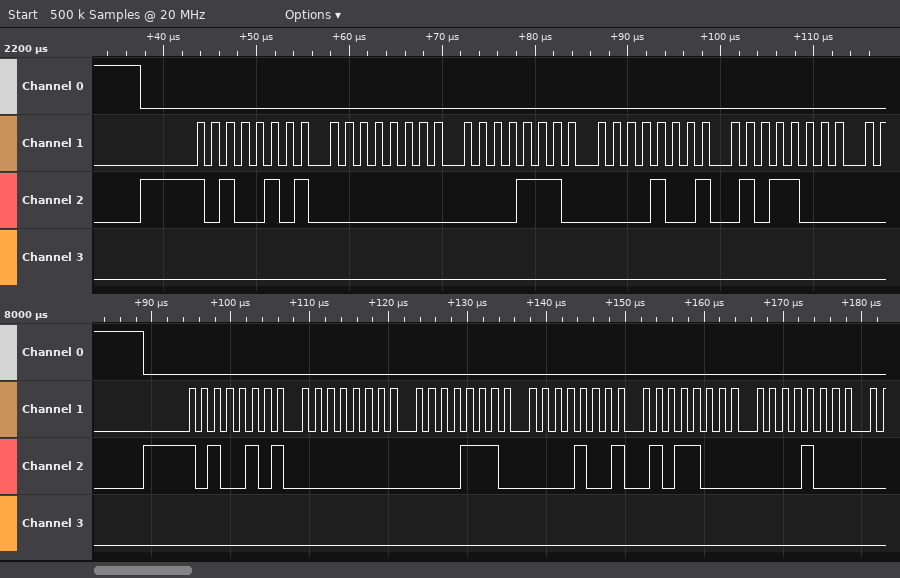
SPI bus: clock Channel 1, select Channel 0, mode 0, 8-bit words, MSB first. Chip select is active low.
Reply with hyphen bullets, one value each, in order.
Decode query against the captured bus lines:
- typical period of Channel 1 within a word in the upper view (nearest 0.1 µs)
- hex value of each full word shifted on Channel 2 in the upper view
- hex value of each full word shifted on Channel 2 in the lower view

- 1.6 µs
- A5, 00, 0E, 09, 58
- A5, 00, 0E, 09, 58, 08
